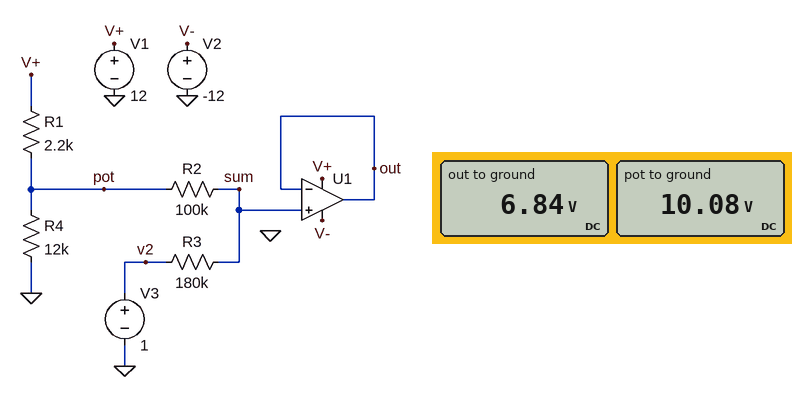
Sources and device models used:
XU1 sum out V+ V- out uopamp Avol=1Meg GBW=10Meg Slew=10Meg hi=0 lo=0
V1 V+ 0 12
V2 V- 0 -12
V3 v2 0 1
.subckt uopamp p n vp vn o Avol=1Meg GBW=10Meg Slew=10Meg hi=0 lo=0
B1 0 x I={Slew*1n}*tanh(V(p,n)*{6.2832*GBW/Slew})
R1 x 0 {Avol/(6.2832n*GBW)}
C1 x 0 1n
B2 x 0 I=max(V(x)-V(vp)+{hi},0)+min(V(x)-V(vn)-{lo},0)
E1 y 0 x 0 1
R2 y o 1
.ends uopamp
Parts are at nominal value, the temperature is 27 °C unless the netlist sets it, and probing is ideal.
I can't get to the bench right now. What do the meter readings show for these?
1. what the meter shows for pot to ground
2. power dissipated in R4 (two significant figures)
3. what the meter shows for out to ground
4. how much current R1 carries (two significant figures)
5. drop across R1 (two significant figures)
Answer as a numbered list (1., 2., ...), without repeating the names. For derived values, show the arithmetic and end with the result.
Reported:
1. 10.08 V
2. (10.08 V)^2 / 12 kΩ = 8.5 mW
3. 6.84 V
4. (12 V - 10.08 V) / 2.2 kΩ = 870 µA
5. 12 V - 10.08 V = 1.9 V
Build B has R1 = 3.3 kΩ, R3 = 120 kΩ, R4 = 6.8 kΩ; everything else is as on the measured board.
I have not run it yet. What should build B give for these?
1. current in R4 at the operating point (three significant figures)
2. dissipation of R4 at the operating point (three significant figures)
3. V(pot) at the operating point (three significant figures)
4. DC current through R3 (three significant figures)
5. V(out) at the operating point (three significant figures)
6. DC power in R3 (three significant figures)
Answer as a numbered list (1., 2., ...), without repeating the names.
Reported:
1. 1.18 mA
2. 9.43 mW
3. 8.01 V
4. 31.9 µA
5. 4.82 V
6. 122 µW
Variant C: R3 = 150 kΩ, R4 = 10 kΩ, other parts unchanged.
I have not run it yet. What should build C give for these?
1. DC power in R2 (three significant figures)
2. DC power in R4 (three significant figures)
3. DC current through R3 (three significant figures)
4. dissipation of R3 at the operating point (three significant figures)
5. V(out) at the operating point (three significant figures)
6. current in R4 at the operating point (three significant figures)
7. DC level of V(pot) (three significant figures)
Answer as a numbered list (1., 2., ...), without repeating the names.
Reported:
1. 123 µW
2. 9.55 mW
3. 35.1 µA
4. 185 µW
5. 6.26 V
6. 977 µA
7. 9.77 V
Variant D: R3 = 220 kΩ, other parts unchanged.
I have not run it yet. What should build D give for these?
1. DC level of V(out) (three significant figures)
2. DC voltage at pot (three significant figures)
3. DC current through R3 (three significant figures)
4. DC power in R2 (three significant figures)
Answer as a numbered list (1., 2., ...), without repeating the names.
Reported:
1. 7.25 V
2. 10.1 V
3. 28.4 µA
4. 80.7 µW
